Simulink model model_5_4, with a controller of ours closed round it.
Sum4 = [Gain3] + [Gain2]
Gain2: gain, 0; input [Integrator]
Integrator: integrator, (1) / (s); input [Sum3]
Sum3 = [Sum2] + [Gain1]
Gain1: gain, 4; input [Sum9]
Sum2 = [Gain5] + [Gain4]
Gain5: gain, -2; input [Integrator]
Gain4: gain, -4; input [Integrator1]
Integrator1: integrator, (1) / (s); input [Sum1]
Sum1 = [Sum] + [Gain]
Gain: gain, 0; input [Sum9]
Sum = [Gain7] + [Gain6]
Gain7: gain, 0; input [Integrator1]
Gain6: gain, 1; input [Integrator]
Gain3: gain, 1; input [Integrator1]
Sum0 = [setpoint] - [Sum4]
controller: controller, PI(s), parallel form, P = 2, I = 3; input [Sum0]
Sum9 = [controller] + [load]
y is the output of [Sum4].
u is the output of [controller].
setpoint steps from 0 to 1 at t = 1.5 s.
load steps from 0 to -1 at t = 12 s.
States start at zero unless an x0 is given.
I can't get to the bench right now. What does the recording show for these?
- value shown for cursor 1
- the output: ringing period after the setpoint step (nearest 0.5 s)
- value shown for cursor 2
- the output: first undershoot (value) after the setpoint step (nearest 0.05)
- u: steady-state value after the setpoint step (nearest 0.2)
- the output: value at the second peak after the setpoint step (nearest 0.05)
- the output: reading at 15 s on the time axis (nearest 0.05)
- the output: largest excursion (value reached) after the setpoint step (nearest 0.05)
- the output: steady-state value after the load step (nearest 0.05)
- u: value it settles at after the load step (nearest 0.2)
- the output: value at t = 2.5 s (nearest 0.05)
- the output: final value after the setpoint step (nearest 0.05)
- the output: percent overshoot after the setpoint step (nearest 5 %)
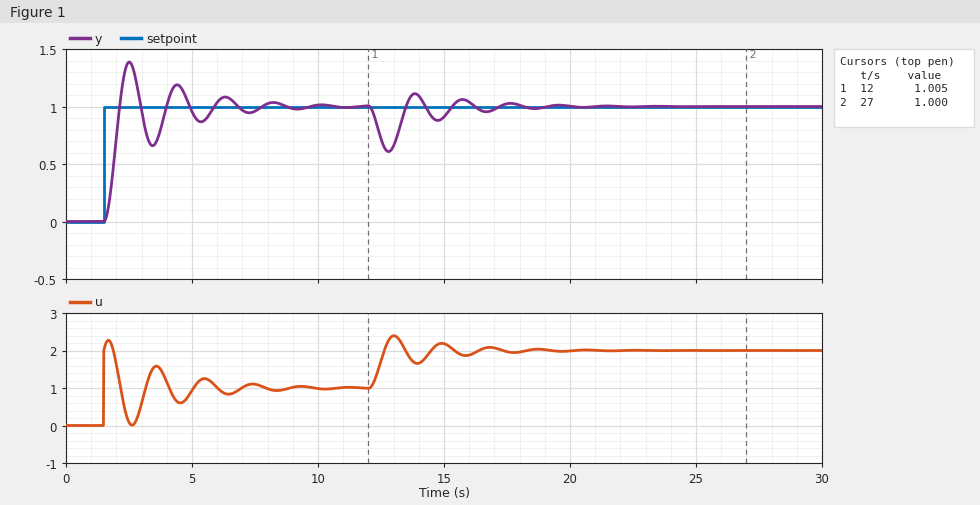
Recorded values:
1.005
2.0 s
1.000
0.65
1.0
1.20
0.90
1.40
1.00
2.0
1.40
1.00
40 %
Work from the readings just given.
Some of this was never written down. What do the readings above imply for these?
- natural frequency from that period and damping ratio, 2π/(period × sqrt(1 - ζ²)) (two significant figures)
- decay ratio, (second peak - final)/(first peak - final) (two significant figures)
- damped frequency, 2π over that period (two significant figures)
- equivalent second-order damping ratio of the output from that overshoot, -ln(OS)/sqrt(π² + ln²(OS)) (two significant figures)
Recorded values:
3.3 rad/s
0.50
3.1 rad/s
0.28
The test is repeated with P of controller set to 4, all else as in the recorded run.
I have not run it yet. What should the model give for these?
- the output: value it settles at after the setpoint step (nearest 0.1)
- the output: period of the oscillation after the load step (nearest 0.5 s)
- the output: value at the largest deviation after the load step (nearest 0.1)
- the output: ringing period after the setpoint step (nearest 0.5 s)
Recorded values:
1.0
1.5 s
0.7
1.5 s
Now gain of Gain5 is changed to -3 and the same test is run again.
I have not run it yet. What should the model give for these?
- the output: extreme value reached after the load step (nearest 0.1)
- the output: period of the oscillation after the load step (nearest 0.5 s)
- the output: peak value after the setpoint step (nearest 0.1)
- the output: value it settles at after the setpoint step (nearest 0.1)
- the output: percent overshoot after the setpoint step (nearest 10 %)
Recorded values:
0.7
2.0 s
1.3
1.0
30 %
